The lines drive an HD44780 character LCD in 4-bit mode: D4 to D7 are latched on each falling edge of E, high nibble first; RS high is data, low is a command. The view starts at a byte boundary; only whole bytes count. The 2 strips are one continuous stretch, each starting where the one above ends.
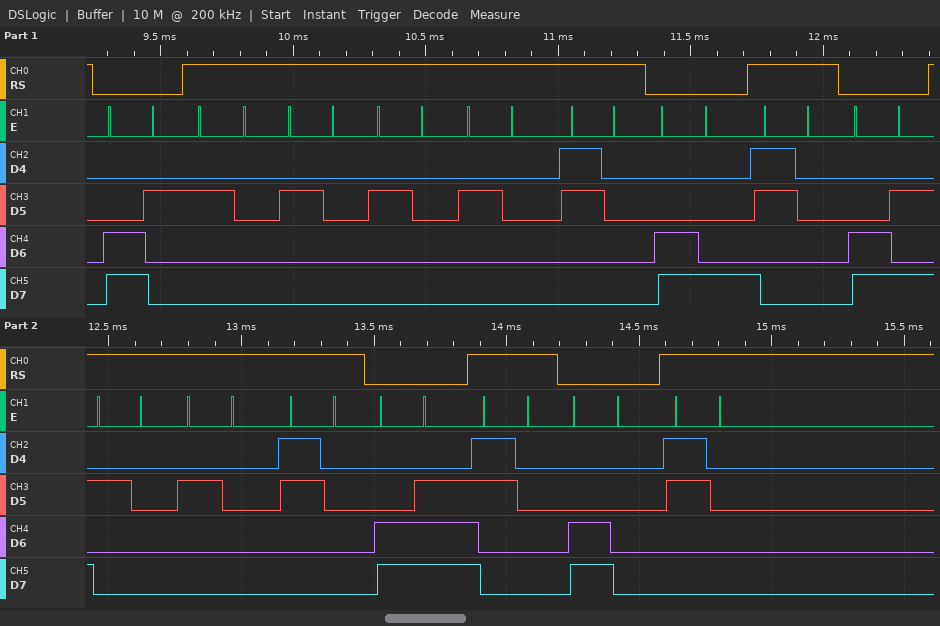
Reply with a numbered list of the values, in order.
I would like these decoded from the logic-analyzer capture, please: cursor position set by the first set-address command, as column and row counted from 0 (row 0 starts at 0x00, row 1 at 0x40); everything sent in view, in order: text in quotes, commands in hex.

1. column 2, row 1
2. 0xC2 "    0" 0xC8 "0" 0xCA "  0" 0xCE "0" 0xC0 "0"
